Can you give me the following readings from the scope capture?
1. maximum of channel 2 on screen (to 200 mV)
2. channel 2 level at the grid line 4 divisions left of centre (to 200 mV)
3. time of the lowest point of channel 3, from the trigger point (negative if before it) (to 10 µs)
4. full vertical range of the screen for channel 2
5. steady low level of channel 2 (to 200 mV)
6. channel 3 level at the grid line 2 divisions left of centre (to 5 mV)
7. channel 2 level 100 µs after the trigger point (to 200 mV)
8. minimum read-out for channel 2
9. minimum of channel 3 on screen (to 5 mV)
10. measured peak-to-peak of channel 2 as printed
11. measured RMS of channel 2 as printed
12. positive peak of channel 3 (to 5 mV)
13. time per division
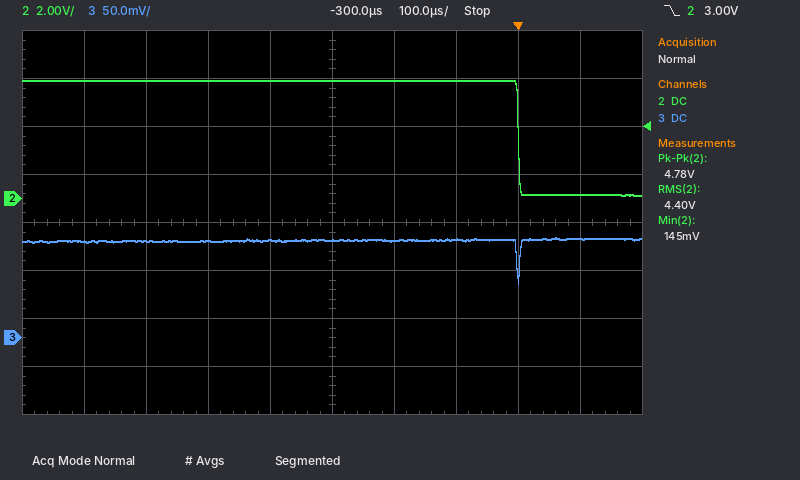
5.0 V
5.0 V
0 µs
16 V
200 mV
100 mV
200 mV
145 mV
55 mV
4.78 V
4.40 V
105 mV
100 µs
